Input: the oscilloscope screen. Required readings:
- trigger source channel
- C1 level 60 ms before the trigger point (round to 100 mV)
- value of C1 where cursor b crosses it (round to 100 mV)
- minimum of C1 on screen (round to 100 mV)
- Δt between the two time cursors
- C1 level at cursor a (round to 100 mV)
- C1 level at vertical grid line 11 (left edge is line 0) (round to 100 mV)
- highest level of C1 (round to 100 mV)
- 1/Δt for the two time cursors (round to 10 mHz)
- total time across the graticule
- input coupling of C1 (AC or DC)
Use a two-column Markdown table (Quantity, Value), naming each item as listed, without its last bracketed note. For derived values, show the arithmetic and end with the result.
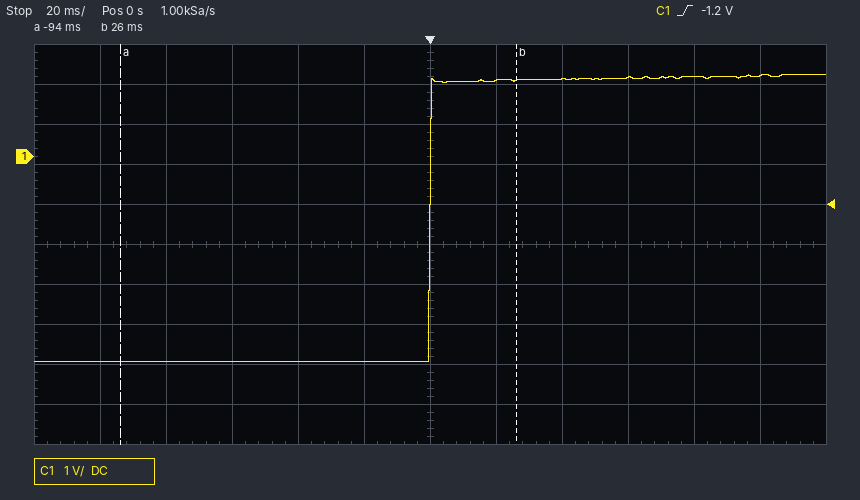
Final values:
| Quantity | Value |
|---|---|
| trigger source channel | C1 |
| C1 level 60 ms before the trigger point | -5.1 V |
| value of C1 where cursor b crosses it | 1.9 V |
| minimum of C1 on screen | -5.1 V |
| Δt between the two time cursors | 26 ms − (-94 ms) = 120 ms |
| C1 level at cursor a | -5.1 V |
| C1 level at vertical grid line 11 (left edge is line 0) | 2.0 V |
| highest level of C1 | 2.0 V |
| 1/Δt for the two time cursors | 1 / 120 ms ≈ 8.33 Hz |
| total time across the graticule | 240 ms |
| input coupling of C1 | DC |
